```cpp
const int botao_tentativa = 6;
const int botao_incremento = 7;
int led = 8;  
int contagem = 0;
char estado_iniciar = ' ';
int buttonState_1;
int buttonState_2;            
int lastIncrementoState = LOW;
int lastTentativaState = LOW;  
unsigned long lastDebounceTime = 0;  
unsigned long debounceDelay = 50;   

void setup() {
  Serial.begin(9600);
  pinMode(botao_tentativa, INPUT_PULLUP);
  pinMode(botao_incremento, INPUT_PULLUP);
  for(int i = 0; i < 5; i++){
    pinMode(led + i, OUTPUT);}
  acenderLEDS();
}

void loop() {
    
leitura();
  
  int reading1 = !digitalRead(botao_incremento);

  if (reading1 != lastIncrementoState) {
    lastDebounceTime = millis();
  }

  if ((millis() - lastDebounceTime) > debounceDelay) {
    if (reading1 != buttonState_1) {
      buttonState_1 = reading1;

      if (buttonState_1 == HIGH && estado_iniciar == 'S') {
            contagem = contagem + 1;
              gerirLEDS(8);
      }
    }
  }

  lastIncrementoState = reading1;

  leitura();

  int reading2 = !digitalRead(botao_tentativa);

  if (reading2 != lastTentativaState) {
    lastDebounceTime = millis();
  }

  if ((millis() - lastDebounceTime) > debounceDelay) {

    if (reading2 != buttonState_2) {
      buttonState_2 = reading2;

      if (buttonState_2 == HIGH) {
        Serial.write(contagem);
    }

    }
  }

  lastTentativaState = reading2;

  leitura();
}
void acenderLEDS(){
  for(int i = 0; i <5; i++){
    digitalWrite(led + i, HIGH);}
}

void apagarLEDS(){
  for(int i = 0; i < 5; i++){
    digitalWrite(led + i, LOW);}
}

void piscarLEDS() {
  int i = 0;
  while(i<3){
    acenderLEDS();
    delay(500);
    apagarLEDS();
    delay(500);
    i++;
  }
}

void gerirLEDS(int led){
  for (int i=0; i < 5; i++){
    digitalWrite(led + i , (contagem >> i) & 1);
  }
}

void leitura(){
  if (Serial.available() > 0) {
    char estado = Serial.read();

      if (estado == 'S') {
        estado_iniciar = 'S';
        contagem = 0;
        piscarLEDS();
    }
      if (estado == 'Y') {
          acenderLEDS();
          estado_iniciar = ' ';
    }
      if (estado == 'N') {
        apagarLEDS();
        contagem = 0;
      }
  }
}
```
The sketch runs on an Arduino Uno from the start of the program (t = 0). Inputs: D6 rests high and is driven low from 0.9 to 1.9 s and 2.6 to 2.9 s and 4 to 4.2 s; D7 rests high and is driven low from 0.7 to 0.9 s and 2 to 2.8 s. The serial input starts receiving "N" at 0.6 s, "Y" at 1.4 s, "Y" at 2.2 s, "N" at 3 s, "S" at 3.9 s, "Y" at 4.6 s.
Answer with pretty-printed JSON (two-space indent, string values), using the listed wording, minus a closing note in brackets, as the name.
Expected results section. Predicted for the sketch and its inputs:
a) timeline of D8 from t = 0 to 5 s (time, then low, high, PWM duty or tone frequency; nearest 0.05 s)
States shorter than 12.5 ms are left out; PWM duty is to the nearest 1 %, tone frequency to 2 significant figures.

{
  "timeline of D8 from t = 0 to 5 s": "0 s high; 0.6 s low; 1.4 s high; 3 s low; 3.9 s high; 4.4 s low; 4.9 s high"
}
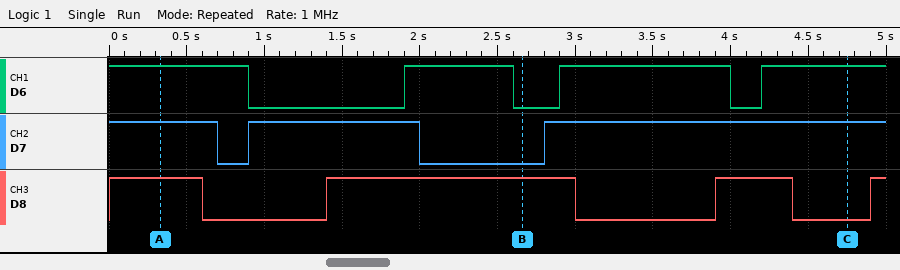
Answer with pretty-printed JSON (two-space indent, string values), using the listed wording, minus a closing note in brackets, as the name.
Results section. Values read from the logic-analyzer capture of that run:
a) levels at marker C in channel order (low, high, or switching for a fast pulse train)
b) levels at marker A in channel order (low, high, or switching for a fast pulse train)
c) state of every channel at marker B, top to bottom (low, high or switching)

{
  "levels at marker C in channel order": "D6 high, D7 high, D8 low",
  "levels at marker A in channel order": "D6 high, D7 high, D8 high",
  "state of every channel at marker B, top to bottom": "D6 low, D7 low, D8 high"
}
